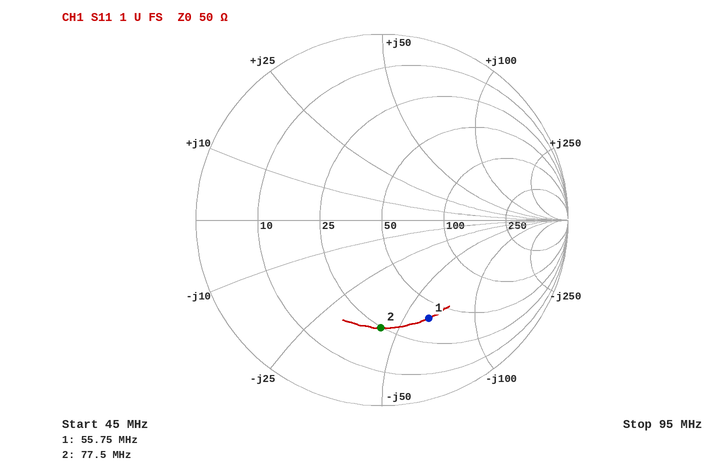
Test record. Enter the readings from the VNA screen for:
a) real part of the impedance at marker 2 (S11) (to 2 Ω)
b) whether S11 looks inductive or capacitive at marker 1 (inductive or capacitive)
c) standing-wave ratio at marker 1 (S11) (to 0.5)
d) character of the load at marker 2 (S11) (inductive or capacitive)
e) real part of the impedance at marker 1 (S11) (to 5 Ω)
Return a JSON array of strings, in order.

["24 Ω", "capacitive", "4.0", "capacitive", "40 Ω"]
